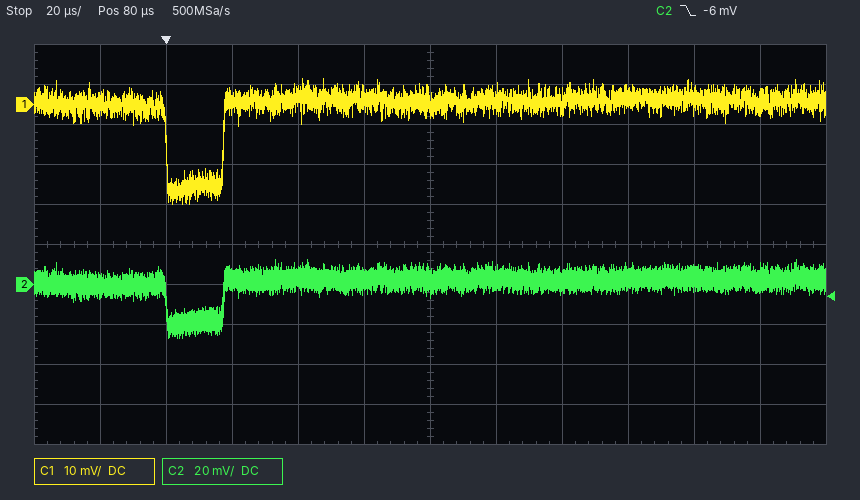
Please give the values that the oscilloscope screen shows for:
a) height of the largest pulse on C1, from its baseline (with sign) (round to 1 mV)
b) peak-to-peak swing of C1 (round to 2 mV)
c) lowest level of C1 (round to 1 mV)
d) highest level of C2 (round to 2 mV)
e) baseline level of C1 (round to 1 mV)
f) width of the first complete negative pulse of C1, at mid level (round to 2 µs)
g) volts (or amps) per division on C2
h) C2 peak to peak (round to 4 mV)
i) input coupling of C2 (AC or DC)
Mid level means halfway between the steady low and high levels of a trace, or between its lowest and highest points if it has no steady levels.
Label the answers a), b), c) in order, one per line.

a) -26 mV
b) 32 mV
c) -25 mV
d) 12 mV
e) 1 mV
f) 18 µs
g) 20 mV
h) 40 mV
i) DC
